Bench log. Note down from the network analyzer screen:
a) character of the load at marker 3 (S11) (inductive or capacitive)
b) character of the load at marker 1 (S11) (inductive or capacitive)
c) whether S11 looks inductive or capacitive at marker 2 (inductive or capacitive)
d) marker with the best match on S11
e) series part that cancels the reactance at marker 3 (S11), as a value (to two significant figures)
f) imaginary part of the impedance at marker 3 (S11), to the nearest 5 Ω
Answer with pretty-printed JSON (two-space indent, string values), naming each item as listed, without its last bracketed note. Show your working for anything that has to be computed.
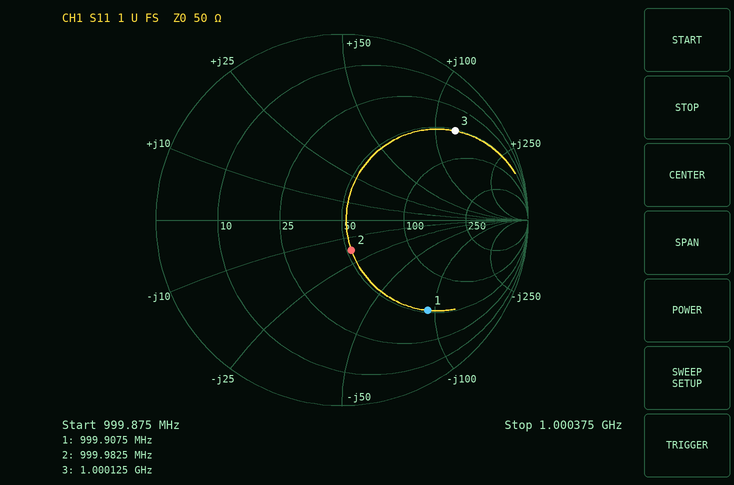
{
  "character of the load at marker 3 (S11)": "inductive",
  "character of the load at marker 1 (S11)": "capacitive",
  "whether S11 looks inductive or capacitive at marker 2": "capacitive",
  "marker with the best match on S11": "marker 2",
  "series part that cancels the reactance at marker 3 (S11), as a value": "C = 1/(2π × 1.000125 GHz × 125 Ω) ≈ 1.3 pF",
  "imaginary part of the impedance at marker 3 (S11), to the nearest 5 Ω": "+125 Ω"
}
